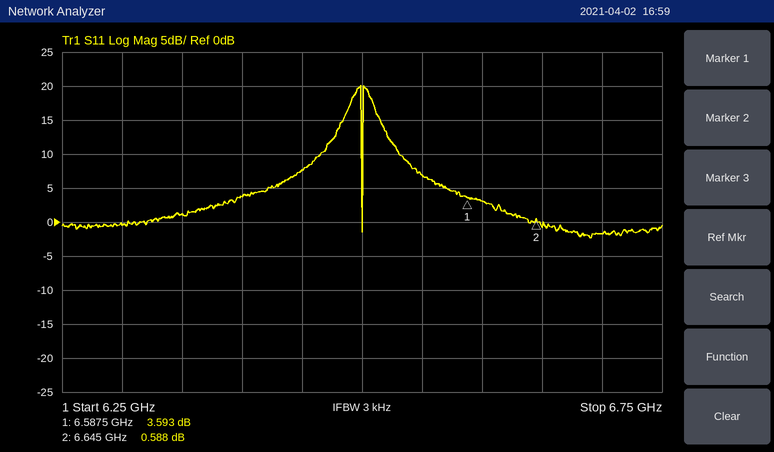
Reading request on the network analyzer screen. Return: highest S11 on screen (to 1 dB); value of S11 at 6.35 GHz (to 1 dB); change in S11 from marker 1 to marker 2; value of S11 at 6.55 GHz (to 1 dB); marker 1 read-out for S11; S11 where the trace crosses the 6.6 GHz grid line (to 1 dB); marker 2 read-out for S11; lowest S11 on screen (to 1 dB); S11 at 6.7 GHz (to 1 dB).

20 dB
1 dB
-3.005 dB
7 dB
3.593 dB
3 dB
0.588 dB
-2 dB
-2 dB
